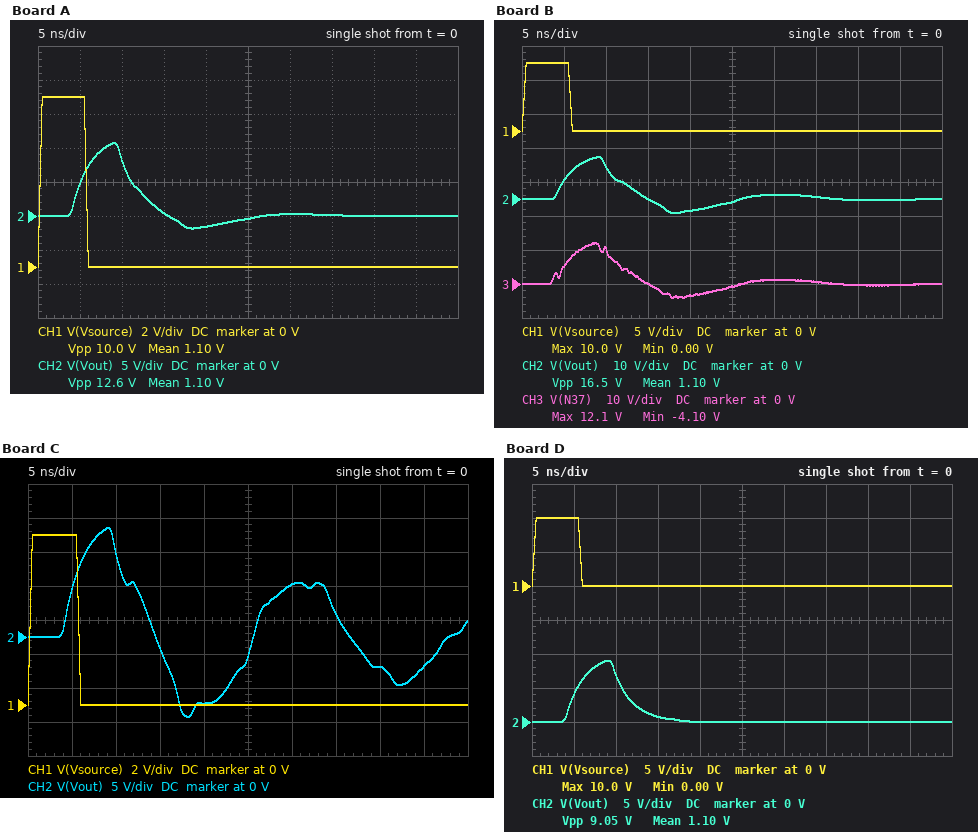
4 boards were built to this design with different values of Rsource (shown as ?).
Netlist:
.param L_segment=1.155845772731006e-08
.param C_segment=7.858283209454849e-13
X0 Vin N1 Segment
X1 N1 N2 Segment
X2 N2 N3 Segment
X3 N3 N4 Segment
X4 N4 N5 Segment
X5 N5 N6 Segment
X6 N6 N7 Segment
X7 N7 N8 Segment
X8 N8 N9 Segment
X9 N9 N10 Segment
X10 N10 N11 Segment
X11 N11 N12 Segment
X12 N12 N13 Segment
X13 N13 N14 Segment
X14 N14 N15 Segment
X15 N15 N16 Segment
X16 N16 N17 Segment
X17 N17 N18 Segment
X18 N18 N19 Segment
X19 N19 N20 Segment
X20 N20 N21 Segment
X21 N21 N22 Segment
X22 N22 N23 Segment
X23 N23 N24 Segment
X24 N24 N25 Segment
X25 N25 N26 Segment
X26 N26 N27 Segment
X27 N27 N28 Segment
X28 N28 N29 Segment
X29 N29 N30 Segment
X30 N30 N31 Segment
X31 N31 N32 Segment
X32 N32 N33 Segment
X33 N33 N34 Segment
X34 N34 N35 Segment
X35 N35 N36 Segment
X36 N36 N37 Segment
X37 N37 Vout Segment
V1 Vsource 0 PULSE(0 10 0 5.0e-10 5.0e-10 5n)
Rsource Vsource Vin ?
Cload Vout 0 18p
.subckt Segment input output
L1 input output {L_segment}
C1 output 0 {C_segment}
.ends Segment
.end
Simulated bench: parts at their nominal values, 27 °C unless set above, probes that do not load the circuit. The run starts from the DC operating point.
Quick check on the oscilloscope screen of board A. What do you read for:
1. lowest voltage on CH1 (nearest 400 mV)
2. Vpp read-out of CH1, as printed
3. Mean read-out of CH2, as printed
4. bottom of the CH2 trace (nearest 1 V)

0 V
10.0 V
1.10 V
-2 V
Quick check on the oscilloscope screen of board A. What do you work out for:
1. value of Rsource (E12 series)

82 Ω
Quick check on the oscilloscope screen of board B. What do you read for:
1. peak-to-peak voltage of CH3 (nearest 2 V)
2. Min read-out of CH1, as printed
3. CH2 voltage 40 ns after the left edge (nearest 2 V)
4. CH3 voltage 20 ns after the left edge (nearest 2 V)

16 V
0.00 V
0 V
-4 V
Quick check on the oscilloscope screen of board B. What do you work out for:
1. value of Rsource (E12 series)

56 Ω
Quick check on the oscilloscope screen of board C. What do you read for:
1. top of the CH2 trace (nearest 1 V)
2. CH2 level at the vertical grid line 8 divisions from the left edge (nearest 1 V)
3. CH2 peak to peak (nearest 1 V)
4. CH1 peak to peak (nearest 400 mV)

16 V
-4 V
28 V
10.0 V
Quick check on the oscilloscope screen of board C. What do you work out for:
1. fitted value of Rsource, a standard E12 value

15 Ω
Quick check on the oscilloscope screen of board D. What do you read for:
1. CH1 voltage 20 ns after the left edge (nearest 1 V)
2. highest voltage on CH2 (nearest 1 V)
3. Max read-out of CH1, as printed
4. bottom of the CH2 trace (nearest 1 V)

0 V
9 V
10.0 V
0 V
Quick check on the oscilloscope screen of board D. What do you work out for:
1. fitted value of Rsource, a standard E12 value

120 Ω
